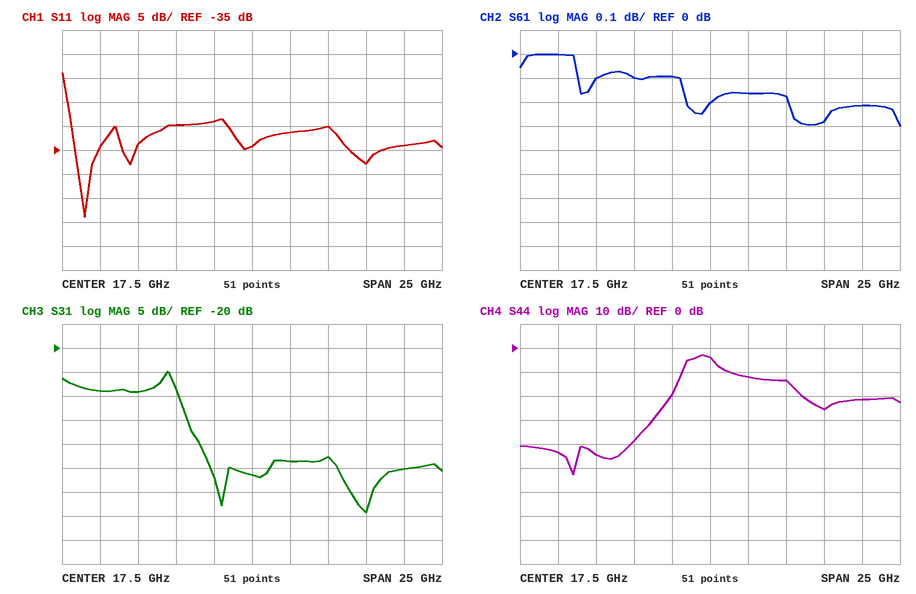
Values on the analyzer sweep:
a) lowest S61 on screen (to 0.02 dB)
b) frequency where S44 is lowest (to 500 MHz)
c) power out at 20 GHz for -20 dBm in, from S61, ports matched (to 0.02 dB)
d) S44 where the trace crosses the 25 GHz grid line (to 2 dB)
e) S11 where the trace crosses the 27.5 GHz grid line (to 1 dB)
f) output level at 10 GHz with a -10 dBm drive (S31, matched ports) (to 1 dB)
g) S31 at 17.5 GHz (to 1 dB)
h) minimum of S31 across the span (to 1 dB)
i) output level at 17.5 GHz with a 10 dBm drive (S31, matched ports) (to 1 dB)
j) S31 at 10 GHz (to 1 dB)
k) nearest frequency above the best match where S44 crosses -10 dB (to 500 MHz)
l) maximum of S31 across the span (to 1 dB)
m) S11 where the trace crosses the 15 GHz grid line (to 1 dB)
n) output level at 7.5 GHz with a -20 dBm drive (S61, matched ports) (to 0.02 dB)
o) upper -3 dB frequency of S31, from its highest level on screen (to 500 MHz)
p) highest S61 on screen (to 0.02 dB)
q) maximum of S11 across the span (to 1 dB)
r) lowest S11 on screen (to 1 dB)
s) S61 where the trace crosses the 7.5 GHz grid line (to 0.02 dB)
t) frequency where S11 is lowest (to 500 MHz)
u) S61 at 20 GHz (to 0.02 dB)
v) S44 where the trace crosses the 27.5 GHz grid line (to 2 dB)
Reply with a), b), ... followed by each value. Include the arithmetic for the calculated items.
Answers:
a) -0.30 dB
b) 8.5 GHz
c) -20 dBm + (-0.16 dB) = -20.16 dBm
d) -26 dB
e) -34 dB
f) -10 dBm + (-29 dB) = -39 dBm
g) -46 dB
h) -54 dB
i) 10 dBm + (-46 dB) = -36 dBm
j) -29 dB
k) 15.5 GHz
l) -25 dB
m) -29 dB
n) -20 dBm + (0.00 dB) = -20.00 dBm
o) 12.5 GHz
p) 0.00 dB
q) -19 dB
r) -49 dB
s) 0.00 dB
t) 6.5 GHz
u) -0.16 dB
v) -22 dB
